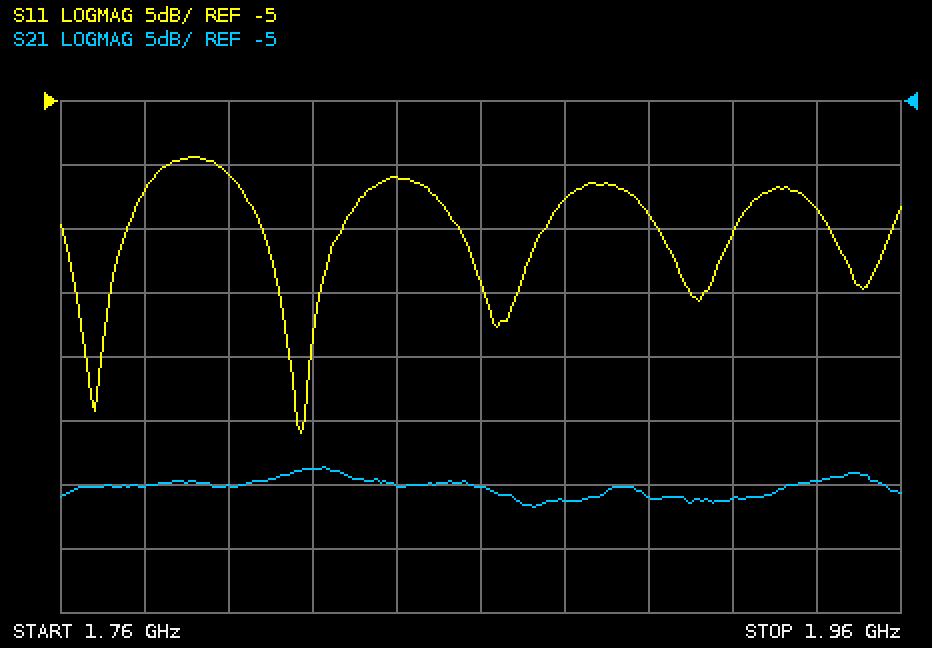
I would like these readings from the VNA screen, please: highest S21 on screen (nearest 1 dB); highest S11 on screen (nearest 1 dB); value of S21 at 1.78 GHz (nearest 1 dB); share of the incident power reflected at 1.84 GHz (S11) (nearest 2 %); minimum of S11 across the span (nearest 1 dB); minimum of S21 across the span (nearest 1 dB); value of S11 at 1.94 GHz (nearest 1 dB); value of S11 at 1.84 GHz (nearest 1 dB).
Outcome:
-34 dB
-9 dB
-35 dB
8 %
-31 dB
-37 dB
-13 dB
-11 dB
